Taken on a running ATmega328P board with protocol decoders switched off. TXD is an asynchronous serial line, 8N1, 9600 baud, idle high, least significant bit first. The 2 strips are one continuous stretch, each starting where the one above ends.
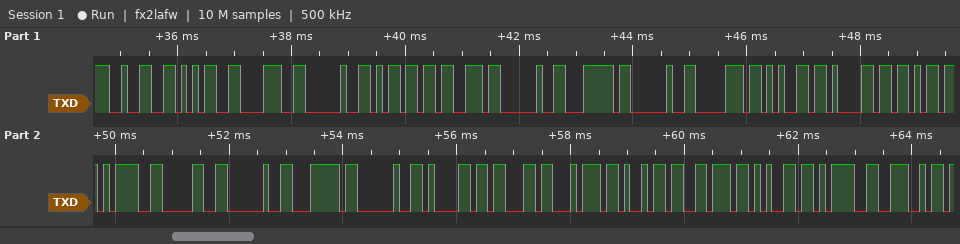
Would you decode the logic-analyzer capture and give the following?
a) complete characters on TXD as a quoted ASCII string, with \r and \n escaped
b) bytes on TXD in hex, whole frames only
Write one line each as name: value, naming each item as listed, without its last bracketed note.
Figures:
complete characters on TXD as a quoted ASCII string, with \r and \n escaped: "258 ms | peak=0 | active=N"
bytes on TXD in hex, whole frames only: 32 35 38 20 6D 73 20 7C 20 70 65 61 6B 3D 30 20 7C 20 61 63 74 69 76 65 3D 4E
